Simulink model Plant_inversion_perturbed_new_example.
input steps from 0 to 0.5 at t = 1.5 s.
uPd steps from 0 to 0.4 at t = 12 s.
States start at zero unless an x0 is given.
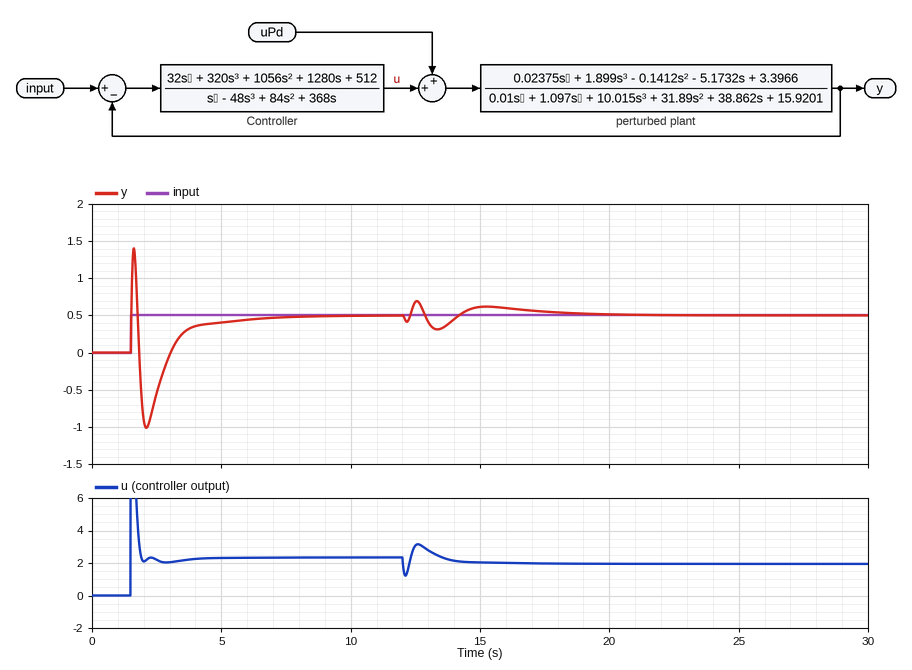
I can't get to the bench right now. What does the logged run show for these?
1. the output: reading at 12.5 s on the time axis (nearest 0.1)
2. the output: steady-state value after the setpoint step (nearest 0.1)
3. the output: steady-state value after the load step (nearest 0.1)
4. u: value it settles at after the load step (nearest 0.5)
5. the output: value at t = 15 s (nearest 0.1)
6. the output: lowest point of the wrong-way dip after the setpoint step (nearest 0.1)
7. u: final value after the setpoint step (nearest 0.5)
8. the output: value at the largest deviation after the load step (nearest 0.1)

0.7
0.5
0.5
2.0
0.6
-1.0
2.5
0.7
